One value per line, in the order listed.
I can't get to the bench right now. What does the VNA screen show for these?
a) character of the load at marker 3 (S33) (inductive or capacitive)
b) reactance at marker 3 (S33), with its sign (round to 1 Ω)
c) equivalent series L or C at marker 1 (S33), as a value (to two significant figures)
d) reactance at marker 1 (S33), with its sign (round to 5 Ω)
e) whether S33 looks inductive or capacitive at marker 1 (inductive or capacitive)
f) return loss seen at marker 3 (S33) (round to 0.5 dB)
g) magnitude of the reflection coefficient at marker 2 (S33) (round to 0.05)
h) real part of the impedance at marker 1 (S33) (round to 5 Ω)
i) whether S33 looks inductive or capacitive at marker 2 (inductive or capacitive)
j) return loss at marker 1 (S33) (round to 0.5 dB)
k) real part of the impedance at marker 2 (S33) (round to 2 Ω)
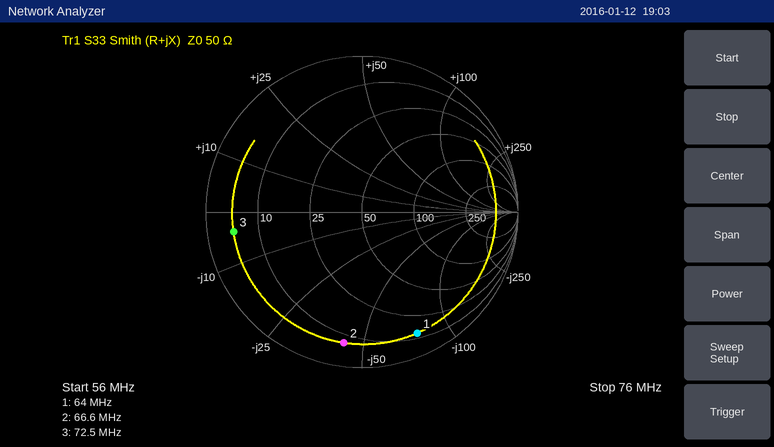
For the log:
capacitive
-4 Ω
33 pF
-75 Ω
capacitive
1.5 dB
0.85
15 Ω
capacitive
1.5 dB
8 Ω
